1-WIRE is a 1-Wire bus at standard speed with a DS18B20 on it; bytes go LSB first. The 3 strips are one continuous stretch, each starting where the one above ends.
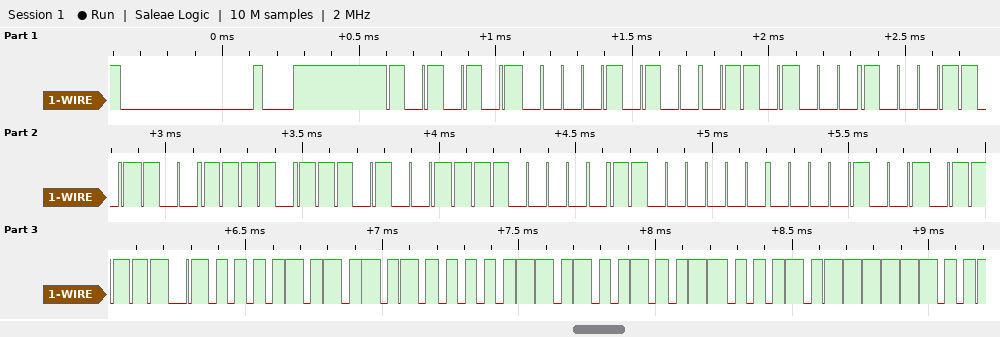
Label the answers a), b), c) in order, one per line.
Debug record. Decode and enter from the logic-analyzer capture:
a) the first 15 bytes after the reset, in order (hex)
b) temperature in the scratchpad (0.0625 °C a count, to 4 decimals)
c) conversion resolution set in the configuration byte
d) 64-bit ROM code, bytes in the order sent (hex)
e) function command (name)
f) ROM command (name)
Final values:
a) 55 28 16 B1 79 97 07 03 90 BE 50 05 4B 46 3F
b) 85.0000 °C
c) 10 bits
d) 28 16 B1 79 97 07 03 90
e) Read Scratchpad
f) Match ROM
